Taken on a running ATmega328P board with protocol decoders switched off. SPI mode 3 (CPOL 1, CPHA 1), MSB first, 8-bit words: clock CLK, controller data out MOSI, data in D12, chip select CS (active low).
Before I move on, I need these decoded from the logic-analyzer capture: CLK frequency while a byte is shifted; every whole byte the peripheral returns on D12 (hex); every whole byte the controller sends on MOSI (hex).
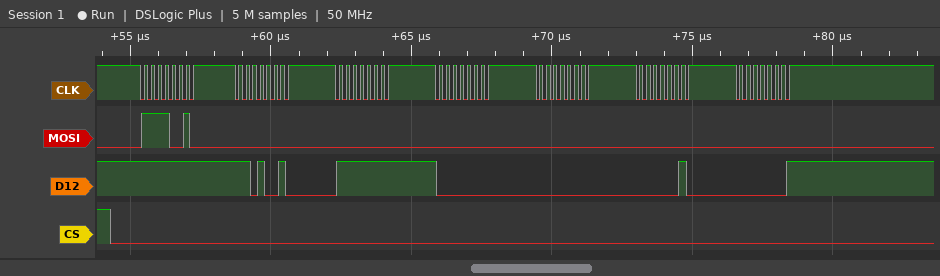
4 MHz
FF D2 FF 00 00 02 01
F2 00 00 00 00 00 00
